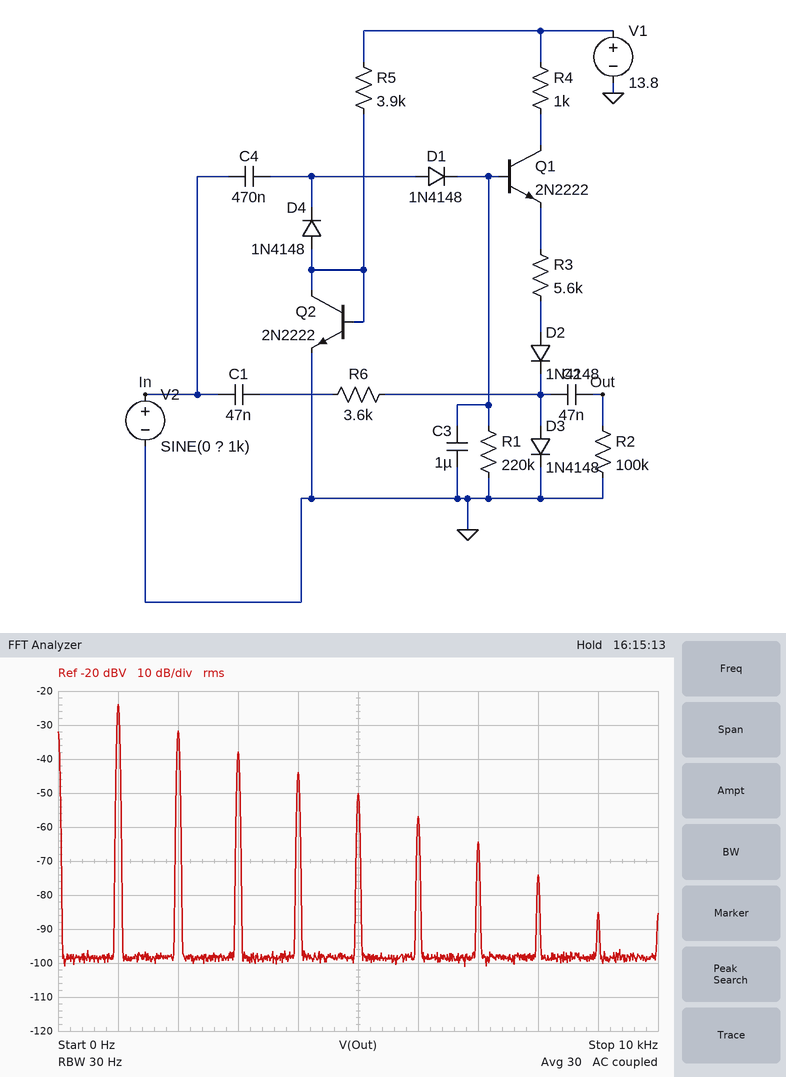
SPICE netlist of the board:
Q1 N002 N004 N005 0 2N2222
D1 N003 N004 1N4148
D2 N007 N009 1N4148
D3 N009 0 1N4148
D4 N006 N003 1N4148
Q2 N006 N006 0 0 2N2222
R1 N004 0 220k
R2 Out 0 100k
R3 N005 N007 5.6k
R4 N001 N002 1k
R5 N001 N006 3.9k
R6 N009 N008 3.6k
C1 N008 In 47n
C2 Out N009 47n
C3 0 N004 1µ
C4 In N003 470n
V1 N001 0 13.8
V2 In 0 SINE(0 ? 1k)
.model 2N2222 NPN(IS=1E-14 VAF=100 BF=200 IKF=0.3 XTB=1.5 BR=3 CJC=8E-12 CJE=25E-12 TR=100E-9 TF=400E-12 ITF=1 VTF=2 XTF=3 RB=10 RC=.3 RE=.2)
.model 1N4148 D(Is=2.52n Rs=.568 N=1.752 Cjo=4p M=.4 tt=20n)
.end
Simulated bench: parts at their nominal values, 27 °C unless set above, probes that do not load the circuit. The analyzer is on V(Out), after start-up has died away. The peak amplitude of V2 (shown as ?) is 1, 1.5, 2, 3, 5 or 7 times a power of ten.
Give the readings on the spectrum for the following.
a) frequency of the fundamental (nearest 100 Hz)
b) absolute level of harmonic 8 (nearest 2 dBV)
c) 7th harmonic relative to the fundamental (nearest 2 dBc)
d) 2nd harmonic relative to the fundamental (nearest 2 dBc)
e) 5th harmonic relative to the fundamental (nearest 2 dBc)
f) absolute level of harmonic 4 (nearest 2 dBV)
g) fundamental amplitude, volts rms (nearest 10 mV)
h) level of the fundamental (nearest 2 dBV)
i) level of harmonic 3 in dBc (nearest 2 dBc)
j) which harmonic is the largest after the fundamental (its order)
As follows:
1.0 kHz
-74 dBV
-40 dBc
-8 dBc
-26 dBc
-44 dBV
60 mV
-24 dBV
-14 dBc
2
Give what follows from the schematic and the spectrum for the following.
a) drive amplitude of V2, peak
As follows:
2 V
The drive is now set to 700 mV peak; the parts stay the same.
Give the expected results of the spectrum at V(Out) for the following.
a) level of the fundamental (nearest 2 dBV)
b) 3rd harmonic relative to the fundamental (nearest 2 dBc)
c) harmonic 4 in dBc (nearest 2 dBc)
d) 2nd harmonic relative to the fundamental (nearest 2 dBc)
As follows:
-12 dBV
-24 dBc
-44 dBc
-18 dBc
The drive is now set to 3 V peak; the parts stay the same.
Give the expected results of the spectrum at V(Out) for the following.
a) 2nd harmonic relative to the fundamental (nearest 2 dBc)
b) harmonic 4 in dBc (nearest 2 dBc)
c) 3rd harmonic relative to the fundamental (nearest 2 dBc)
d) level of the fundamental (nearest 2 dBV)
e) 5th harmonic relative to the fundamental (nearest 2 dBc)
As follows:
-12 dBc
-28 dBc
-20 dBc
-28 dBV
-36 dBc
